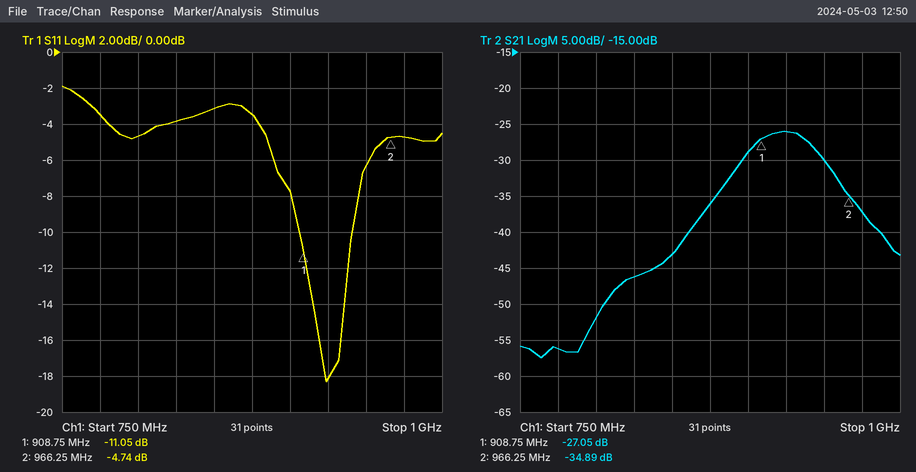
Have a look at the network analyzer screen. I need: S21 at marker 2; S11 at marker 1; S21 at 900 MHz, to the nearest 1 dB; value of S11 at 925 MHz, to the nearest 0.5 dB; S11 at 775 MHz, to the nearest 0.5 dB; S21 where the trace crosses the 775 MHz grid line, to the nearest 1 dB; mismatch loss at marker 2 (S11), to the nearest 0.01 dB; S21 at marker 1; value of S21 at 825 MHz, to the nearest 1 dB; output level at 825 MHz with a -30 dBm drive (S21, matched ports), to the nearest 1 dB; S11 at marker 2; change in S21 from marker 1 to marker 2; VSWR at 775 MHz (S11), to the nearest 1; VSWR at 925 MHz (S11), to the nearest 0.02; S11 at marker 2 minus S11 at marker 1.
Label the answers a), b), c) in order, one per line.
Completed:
a) -34.89 dB
b) -11.05 dB
c) -29 dB
d) -18.0 dB
e) -3.5 dB
f) -56 dB
g) 1.78 dB
h) -27.05 dB
i) -46 dB
j) -76 dBm
k) -4.74 dB
l) -7.84 dB
m) 5
n) 1.28
o) 6.31 dB
